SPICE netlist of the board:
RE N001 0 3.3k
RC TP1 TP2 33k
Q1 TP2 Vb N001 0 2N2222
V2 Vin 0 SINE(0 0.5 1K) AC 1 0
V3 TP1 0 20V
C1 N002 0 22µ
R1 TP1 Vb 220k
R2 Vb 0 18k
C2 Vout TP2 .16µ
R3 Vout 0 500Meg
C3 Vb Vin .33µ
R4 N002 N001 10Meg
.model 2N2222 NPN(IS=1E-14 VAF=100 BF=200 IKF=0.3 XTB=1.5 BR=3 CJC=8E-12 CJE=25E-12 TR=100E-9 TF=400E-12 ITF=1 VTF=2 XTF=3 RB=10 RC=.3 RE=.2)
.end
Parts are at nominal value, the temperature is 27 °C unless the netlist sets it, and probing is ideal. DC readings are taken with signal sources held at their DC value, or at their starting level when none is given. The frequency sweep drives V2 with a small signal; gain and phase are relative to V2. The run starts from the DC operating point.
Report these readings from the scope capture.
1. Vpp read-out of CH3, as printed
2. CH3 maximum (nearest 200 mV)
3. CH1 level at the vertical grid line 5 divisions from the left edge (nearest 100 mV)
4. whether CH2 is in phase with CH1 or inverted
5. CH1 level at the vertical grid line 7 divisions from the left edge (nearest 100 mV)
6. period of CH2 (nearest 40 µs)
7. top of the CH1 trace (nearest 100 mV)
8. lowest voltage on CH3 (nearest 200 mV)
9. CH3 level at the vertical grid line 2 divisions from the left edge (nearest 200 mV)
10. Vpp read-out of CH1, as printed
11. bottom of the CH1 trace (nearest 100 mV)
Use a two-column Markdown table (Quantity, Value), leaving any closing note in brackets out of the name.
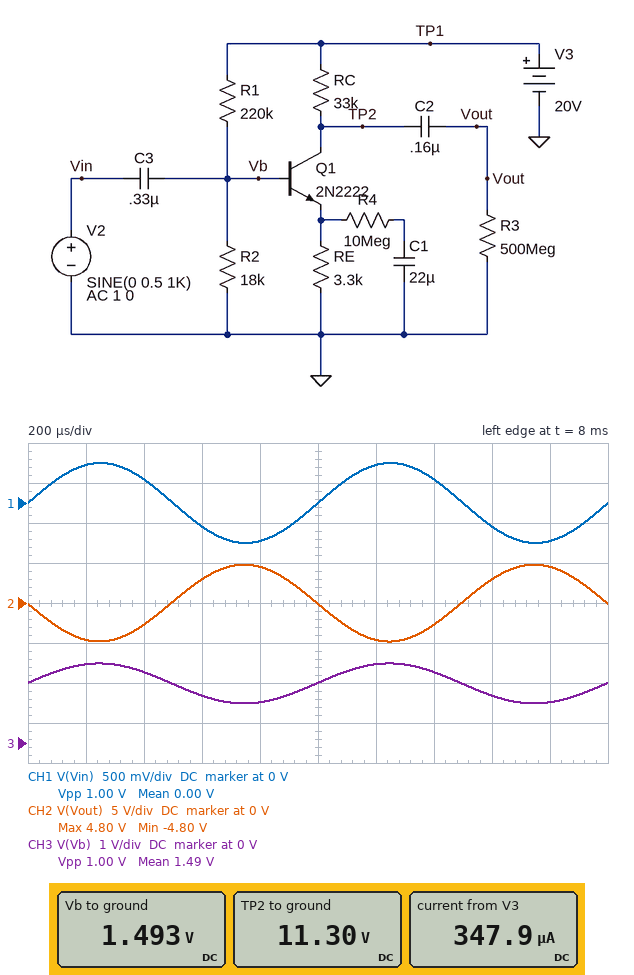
| Quantity | Value |
|---|---|
| Vpp read-out of CH3, as printed | 1.00 V |
| CH3 maximum | 2.0 V |
| CH1 level at the vertical grid line 5 divisions from the left edge | 0 V |
| whether CH2 is in phase with CH1 or inverted | inverted |
| CH1 level at the vertical grid line 7 divisions from the left edge | 300 mV |
| period of CH2 | 1.00 ms |
| top of the CH1 trace | 500 mV |
| lowest voltage on CH3 | 1.0 V |
| CH3 level at the vertical grid line 2 divisions from the left edge | 1.8 V |
| Vpp read-out of CH1, as printed | 1.00 V |
| bottom of the CH1 trace | -500 mV |
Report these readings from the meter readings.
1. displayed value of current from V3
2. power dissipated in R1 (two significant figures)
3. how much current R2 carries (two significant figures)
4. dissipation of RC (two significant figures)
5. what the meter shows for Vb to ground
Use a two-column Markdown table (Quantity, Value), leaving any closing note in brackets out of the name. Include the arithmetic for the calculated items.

| Quantity | Value |
|---|---|
| displayed value of current from V3 | 347.9 µA |
| power dissipated in R1 | (20 V - 1.493 V)^2 / 220 kΩ = 1.6 mW |
| how much current R2 carries | (1.493 V) / 18 kΩ = 83 µA |
| dissipation of RC | (20 V - 11.3 V)^2 / 33 kΩ = 2.3 mW |
| what the meter shows for Vb to ground | 1.493 V |
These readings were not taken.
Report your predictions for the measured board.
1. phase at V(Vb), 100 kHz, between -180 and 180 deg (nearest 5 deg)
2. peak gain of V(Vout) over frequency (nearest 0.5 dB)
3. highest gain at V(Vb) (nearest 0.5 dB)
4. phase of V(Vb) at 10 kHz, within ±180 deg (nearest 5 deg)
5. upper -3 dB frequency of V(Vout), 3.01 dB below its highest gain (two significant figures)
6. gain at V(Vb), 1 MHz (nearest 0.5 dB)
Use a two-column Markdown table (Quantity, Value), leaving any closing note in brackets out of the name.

| Quantity | Value |
|---|---|
| phase at V(Vb), 100 kHz, between -180 and 180 deg | 0 deg |
| peak gain of V(Vout) over frequency | 19.5 dB |
| highest gain at V(Vb) | 0 dB |
| phase of V(Vb) at 10 kHz, within ±180 deg | 0 deg |
| upper -3 dB frequency of V(Vout), 3.01 dB below its highest gain | 1.5 MHz |
| gain at V(Vb), 1 MHz | 0 dB |
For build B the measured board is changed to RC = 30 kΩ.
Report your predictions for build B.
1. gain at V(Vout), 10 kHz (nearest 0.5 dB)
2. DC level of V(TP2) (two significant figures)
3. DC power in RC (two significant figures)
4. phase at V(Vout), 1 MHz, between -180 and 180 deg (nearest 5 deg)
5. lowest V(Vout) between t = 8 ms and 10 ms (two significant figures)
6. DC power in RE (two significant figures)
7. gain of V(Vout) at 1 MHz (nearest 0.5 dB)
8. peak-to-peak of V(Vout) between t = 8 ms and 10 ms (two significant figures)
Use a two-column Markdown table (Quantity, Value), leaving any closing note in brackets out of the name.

| Quantity | Value |
|---|---|
| gain at V(Vout), 10 kHz | 19.0 dB |
| DC level of V(TP2) | 12 V |
| DC power in RC | 2.1 mW |
| phase at V(Vout), 1 MHz, between -180 and 180 deg | 145 deg |
| lowest V(Vout) between t = 8 ms and 10 ms | -4.4 V |
| DC power in RE | 230 µW |
| gain of V(Vout) at 1 MHz | 17.5 dB |
| peak-to-peak of V(Vout) between t = 8 ms and 10 ms | 8.7 V |
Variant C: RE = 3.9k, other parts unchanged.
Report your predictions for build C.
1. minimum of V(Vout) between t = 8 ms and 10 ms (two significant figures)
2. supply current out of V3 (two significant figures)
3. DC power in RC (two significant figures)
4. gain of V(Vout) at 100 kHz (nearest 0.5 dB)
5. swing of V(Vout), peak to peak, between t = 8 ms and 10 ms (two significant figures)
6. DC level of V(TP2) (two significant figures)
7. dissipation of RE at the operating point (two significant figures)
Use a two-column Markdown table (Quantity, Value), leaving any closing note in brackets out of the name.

| Quantity | Value |
|---|---|
| minimum of V(Vout) between t = 8 ms and 10 ms | -4.1 V |
| supply current out of V3 | 310 µA |
| DC power in RC | 1.7 mW |
| gain of V(Vout) at 100 kHz | 18.0 dB |
| swing of V(Vout), peak to peak, between t = 8 ms and 10 ms | 8.1 V |
| DC level of V(TP2) | 13 V |
| dissipation of RE at the operating point | 200 µW |
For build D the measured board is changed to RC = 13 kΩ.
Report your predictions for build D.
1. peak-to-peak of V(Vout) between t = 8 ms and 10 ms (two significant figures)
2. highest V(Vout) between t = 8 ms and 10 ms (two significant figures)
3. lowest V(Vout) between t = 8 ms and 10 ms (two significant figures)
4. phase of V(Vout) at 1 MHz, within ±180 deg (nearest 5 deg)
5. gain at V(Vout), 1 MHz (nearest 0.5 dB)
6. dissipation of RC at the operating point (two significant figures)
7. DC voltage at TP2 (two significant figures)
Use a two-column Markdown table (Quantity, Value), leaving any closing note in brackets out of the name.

| Quantity | Value |
|---|---|
| peak-to-peak of V(Vout) between t = 8 ms and 10 ms | 3.8 V |
| highest V(Vout) between t = 8 ms and 10 ms | 1.9 V |
| lowest V(Vout) between t = 8 ms and 10 ms | -1.9 V |
| phase of V(Vout) at 1 MHz, within ±180 deg | 160 deg |
| gain at V(Vout), 1 MHz | 11.5 dB |
| dissipation of RC at the operating point | 910 µW |
| DC voltage at TP2 | 17 V |
